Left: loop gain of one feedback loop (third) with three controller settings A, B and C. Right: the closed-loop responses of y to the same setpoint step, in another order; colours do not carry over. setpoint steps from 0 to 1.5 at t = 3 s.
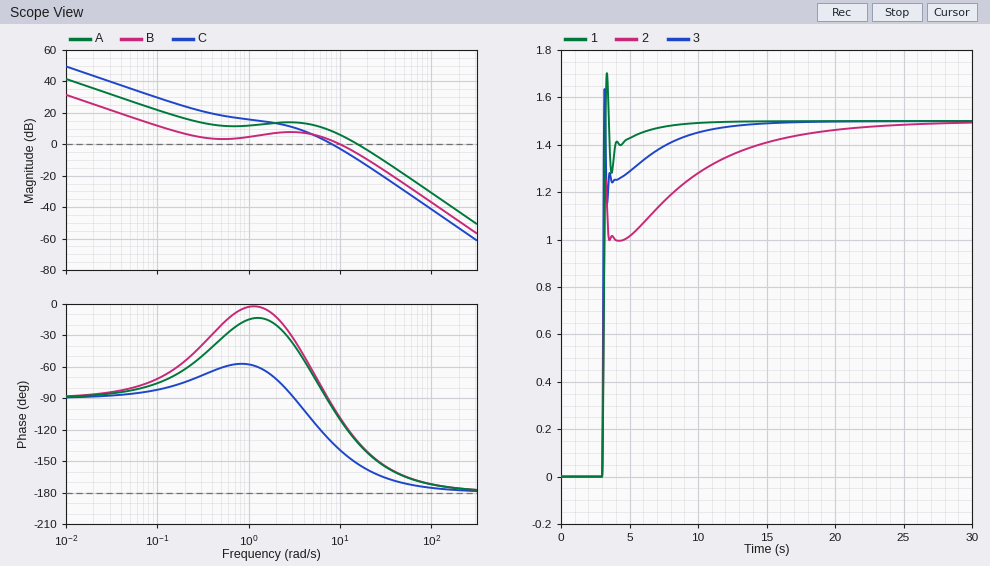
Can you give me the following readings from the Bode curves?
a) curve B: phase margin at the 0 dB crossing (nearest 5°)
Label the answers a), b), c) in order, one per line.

a) 70°
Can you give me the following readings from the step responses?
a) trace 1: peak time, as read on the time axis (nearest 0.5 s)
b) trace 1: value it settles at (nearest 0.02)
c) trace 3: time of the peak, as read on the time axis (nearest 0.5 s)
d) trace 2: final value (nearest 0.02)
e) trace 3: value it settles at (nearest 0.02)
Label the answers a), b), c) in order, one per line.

a) 3.5 s
b) 1.50
c) 3.0 s
d) 1.50
e) 1.50
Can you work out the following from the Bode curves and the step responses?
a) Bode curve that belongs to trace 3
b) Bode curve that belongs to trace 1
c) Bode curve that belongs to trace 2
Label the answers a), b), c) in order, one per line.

a) A
b) C
c) B
